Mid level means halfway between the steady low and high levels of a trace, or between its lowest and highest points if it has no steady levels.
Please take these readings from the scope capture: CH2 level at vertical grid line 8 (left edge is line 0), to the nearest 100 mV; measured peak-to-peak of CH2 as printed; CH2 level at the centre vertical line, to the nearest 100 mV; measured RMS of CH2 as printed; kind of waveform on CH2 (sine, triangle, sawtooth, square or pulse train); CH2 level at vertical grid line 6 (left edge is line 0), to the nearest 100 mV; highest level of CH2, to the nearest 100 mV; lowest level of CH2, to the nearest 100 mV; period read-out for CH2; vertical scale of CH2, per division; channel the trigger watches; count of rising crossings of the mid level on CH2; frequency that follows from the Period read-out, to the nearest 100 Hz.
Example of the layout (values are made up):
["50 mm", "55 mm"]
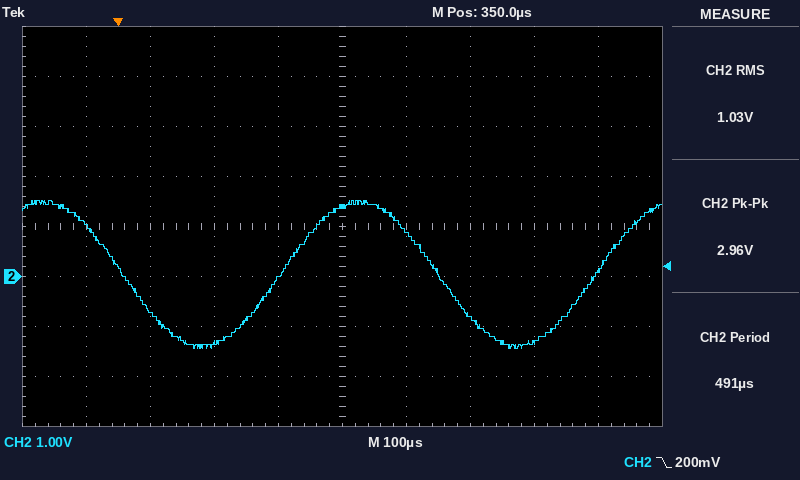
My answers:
["-1.3 V", "2.96 V", "1.4 V", "1.03 V", "sine", "900 mV", "1.5 V", "-1.4 V", "491 µs", "1 V", "CH2", "2", "2.0 kHz"]
